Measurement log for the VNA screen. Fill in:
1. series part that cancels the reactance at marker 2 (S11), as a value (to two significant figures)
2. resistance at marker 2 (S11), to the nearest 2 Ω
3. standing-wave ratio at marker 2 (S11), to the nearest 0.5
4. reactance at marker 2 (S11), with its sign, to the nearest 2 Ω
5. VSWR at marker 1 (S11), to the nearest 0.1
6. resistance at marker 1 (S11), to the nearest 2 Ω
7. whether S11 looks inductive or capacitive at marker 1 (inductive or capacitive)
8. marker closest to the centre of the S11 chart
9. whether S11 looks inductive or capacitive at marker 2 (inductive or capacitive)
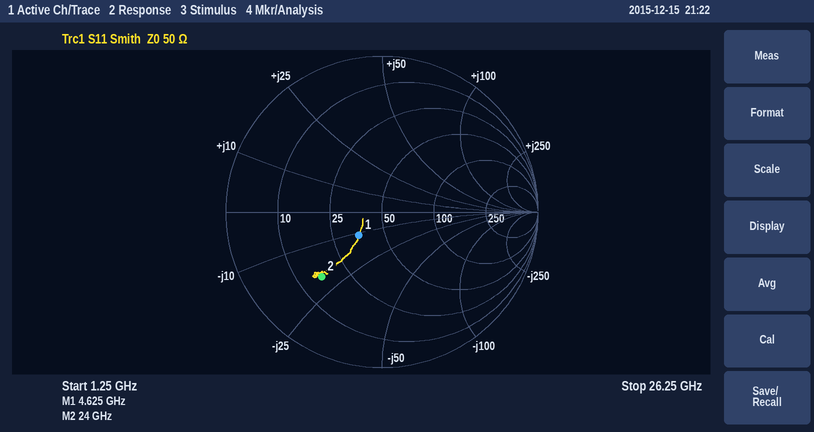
130 pH
16 Ω
3.5
-20 Ω
1.5
36 Ω
capacitive
marker 1
capacitive
